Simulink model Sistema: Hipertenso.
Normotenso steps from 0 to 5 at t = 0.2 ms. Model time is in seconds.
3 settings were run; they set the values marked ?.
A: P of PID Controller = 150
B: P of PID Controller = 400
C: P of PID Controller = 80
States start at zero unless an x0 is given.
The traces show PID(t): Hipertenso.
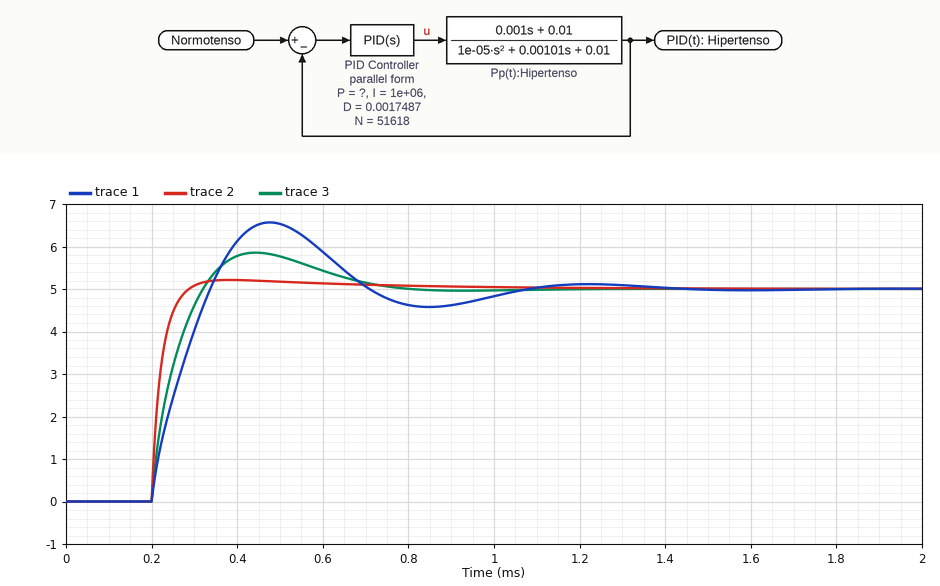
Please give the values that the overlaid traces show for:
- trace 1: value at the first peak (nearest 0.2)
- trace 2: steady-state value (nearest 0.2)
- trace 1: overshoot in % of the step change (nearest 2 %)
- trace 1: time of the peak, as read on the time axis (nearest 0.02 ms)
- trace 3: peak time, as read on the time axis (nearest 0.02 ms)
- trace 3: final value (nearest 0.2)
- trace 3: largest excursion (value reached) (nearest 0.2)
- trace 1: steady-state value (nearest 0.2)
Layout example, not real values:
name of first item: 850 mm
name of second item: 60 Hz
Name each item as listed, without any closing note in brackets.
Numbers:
trace 1: value at the first peak: 6.6
trace 2: steady-state value: 5.0
trace 1: overshoot in % of the step change: 32 %
trace 1: time of the peak, as read on the time axis: 0.48 ms
trace 3: peak time, as read on the time axis: 0.44 ms
trace 3: final value: 5.0
trace 3: largest excursion (value reached): 5.8
trace 1: steady-state value: 5.0
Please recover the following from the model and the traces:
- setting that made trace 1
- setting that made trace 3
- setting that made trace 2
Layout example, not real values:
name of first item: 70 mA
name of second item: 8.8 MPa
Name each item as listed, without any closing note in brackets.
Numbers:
setting that made trace 1: C
setting that made trace 3: A
setting that made trace 2: B
